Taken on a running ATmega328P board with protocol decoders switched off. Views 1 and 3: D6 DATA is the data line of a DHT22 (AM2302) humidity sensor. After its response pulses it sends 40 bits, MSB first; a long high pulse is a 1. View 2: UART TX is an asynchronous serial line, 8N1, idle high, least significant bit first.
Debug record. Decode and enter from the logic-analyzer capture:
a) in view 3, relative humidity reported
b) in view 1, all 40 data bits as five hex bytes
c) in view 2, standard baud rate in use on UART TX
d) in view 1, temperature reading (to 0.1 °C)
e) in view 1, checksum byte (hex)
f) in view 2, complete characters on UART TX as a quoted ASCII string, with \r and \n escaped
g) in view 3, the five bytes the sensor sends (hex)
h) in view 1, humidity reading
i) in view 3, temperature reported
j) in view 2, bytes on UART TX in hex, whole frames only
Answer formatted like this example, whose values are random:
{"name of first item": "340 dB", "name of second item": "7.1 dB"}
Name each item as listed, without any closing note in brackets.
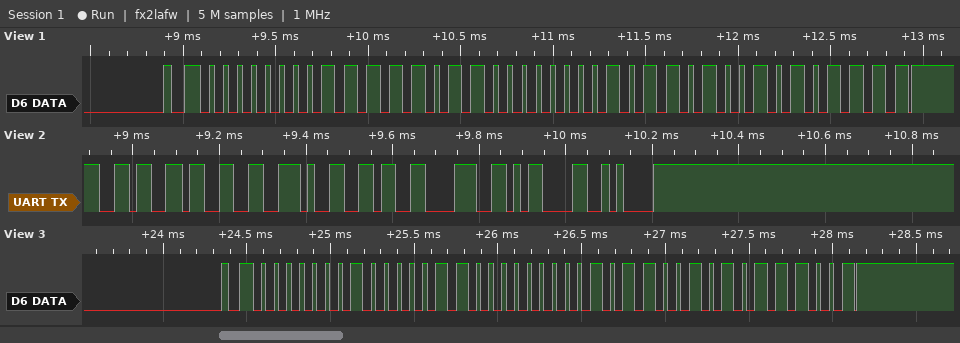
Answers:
{"in view 3, relative humidity reported": "26.2 %", "in view 1, all 40 data bits as five hex bytes": "00 FB 00 B4 AF", "in view 2, standard baud rate in use on UART TX": "57600 baud", "in view 1, temperature reading": "18.0 °C", "in view 1, checksum byte": "0xAF", "in view 2, complete characters on UART TX as a quoted ASCII string, with \\r and \\n escaped": "\"63.68\\r\\n\"", "in view 3, the five bytes the sensor sends": "01 06 00 B2 B9", "in view 1, humidity reading": "25.1 %", "in view 3, temperature reported": "17.8 °C", "in view 2, bytes on UART TX in hex, whole frames only": "36 33 2E 36 38 0D 0A"}
